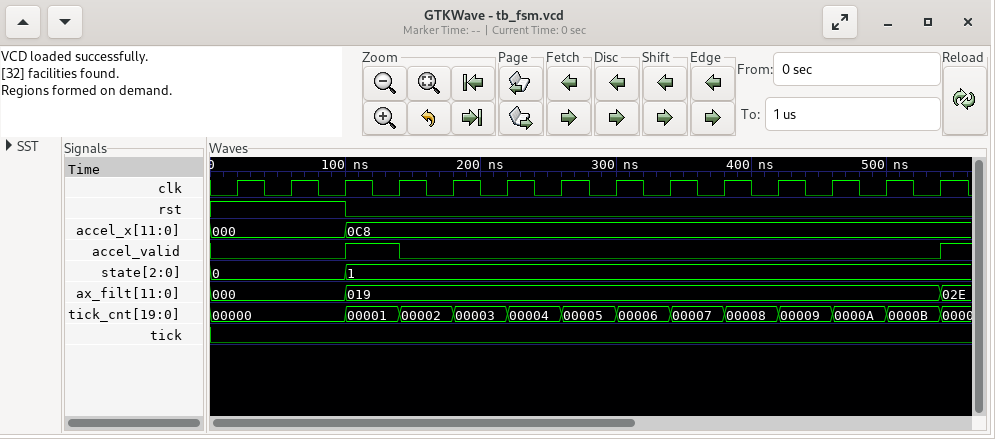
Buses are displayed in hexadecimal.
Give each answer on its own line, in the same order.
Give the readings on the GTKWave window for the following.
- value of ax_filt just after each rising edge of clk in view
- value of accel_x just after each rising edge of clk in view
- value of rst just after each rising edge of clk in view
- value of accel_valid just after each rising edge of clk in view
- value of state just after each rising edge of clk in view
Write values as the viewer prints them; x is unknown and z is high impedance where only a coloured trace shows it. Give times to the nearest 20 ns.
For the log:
000, 000, 019, 019, 019, 019, 019, 019, 019, 019, 019, 019, 019, 02E
000, 000, 0C8, 0C8, 0C8, 0C8, 0C8, 0C8, 0C8, 0C8, 0C8, 0C8, 0C8, 0C8
1 1 0 0 0 0 0 0 0 0 0 0 0 0
0 0 1 0 0 0 0 0 0 0 0 0 0 1
0, 0, 1, 1, 1, 1, 1, 1, 1, 1, 1, 1, 1, 1
